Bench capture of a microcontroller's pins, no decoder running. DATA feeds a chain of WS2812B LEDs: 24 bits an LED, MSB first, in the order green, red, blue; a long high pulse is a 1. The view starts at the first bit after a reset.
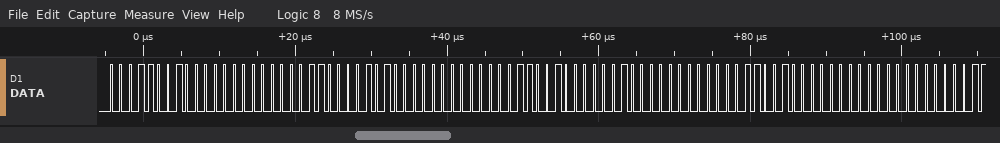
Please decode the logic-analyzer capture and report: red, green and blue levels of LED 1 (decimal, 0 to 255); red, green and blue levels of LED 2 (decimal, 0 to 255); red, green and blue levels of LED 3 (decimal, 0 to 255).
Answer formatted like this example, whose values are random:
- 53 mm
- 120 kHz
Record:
- 0, 25, 6
- 0, 20, 25
- 0, 2, 25
